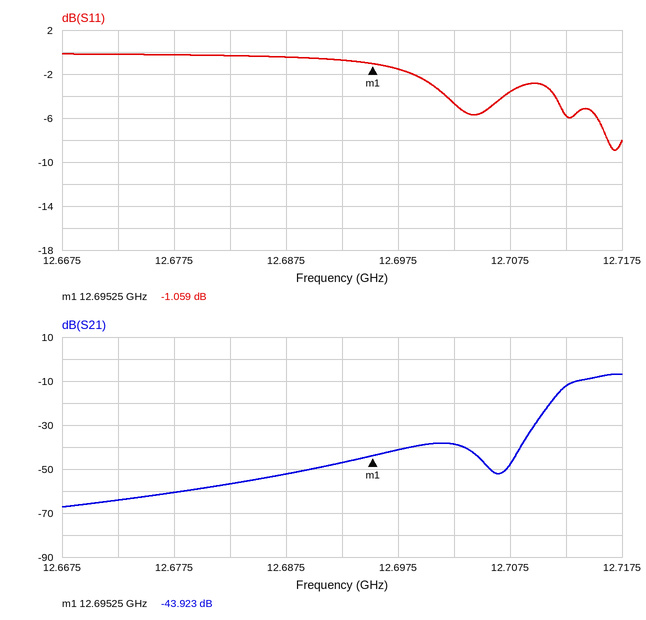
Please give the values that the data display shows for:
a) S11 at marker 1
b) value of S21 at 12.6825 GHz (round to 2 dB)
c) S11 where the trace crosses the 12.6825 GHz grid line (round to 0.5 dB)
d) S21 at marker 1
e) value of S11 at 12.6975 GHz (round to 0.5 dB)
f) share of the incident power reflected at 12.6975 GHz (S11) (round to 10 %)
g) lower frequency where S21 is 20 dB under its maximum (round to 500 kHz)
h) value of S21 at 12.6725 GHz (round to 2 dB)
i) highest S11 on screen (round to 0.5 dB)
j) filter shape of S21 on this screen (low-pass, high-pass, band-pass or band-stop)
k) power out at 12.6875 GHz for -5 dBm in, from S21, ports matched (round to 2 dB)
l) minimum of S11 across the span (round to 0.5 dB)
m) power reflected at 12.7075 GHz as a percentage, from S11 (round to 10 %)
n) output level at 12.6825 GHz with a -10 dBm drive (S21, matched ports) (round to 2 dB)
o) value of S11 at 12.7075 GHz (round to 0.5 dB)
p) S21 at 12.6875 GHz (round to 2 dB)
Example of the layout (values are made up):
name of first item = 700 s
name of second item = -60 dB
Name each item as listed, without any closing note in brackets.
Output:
S11 at marker 1 = -1.059 dB
value of S21 at 12.6825 GHz = -56 dB
S11 where the trace crosses the 12.6825 GHz grid line = -0.5 dB
S21 at marker 1 = -43.923 dB
value of S11 at 12.6975 GHz = -1.5 dB
share of the incident power reflected at 12.6975 GHz (S11) = 70 %
lower frequency where S21 is 20 dB under its maximum = 12.7100 GHz
value of S21 at 12.6725 GHz = -64 dB
highest S11 on screen = 0.0 dB
filter shape of S21 on this screen = high-pass
power out at 12.6875 GHz for -5 dBm in, from S21, ports matched = -58 dBm
minimum of S11 across the span = -9.0 dB
power reflected at 12.7075 GHz as a percentage, from S11 = 40 %
output level at 12.6825 GHz with a -10 dBm drive (S21, matched ports) = -66 dBm
value of S11 at 12.7075 GHz = -3.5 dB
S21 at 12.6875 GHz = -52 dB
